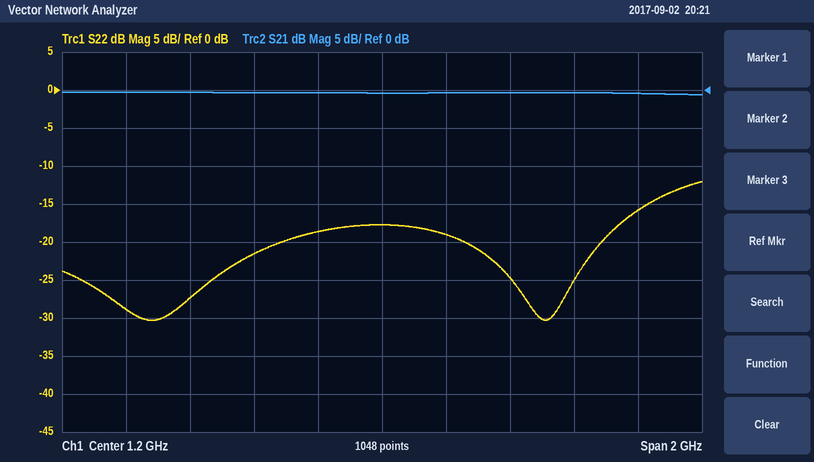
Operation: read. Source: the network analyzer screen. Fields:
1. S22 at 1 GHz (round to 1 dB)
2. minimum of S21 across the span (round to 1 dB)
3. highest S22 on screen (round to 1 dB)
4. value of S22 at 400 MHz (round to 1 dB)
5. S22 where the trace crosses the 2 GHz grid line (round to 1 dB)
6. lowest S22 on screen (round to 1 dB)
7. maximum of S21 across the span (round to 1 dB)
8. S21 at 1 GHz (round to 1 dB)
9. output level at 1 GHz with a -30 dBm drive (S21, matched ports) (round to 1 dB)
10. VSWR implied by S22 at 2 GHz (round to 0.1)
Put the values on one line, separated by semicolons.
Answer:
-19 dB; -1 dB; -12 dB; -29 dB; -16 dB; -30 dB; 0 dB; 0 dB; -30 dBm; 1.4
